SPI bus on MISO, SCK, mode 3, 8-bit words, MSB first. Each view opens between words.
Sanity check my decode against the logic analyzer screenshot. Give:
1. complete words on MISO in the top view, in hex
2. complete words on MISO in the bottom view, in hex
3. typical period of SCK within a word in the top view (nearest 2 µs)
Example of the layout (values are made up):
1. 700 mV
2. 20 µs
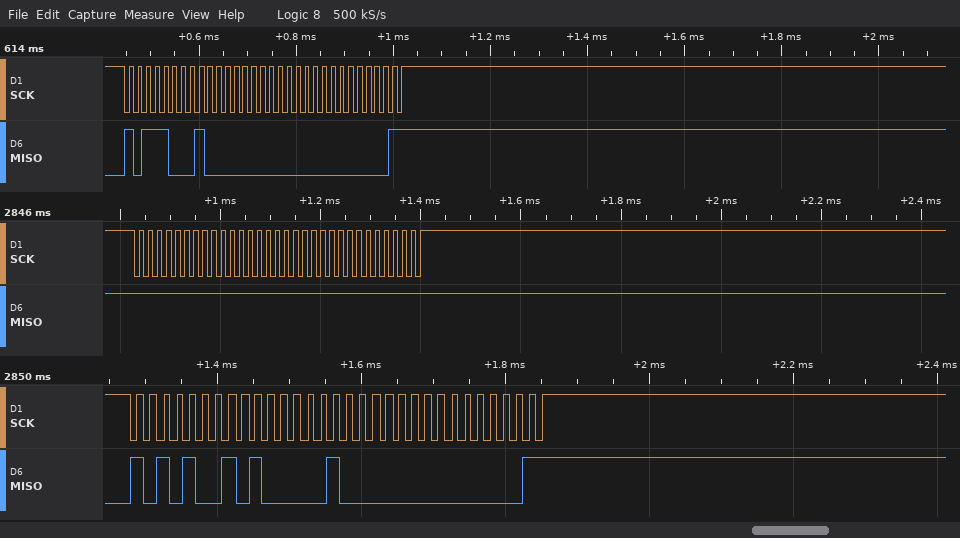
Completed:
1. B8, 80, 00, 03
2. A9, 41, 00, 03
3. 18 µs
